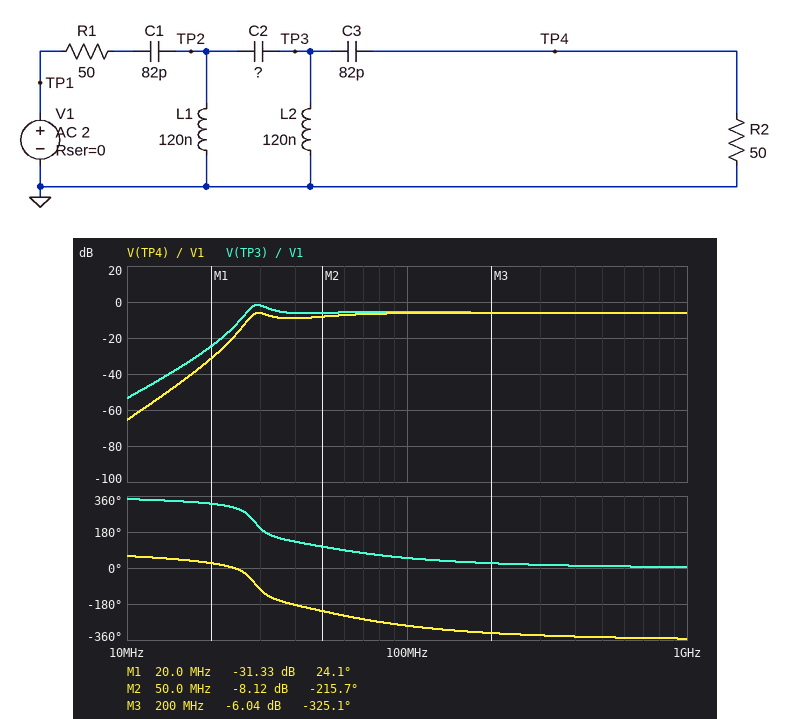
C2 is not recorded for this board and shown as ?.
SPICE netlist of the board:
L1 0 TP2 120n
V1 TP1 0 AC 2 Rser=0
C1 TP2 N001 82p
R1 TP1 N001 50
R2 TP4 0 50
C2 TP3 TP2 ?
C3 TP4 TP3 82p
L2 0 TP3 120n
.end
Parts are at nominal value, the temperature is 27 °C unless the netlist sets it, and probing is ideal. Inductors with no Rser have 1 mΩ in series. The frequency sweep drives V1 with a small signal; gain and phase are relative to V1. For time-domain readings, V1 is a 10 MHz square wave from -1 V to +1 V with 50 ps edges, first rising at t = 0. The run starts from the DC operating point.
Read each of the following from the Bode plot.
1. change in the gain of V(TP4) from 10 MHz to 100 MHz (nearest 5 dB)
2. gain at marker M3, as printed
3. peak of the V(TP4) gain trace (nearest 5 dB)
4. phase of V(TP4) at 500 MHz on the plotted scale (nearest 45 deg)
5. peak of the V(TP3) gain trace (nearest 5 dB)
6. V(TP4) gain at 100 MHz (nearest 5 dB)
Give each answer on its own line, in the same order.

60 dB
-6.04 dB
-5 dB
-360 deg
0 dB
-5 dB
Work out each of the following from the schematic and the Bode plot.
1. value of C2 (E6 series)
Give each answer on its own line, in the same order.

100 pF
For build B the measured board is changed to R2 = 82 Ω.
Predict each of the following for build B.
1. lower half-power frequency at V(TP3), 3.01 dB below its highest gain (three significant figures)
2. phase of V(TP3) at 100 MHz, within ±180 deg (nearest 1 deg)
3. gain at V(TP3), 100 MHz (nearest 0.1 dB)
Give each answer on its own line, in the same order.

27.7 MHz
59 deg
-4.5 dB
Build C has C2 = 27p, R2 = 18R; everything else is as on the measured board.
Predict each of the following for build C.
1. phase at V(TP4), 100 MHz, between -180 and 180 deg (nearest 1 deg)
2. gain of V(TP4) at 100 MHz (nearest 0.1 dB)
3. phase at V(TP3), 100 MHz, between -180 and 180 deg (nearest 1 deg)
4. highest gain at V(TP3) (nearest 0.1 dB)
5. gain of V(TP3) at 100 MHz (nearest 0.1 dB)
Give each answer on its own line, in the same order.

95 deg
-12.5 dB
48 deg
-3.7 dB
-9.2 dB
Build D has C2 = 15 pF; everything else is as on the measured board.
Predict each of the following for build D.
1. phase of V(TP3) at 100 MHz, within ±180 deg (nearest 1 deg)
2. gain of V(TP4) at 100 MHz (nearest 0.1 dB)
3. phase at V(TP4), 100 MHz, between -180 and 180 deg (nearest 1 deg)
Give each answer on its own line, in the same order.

96 deg
-7.7 dB
118 deg
